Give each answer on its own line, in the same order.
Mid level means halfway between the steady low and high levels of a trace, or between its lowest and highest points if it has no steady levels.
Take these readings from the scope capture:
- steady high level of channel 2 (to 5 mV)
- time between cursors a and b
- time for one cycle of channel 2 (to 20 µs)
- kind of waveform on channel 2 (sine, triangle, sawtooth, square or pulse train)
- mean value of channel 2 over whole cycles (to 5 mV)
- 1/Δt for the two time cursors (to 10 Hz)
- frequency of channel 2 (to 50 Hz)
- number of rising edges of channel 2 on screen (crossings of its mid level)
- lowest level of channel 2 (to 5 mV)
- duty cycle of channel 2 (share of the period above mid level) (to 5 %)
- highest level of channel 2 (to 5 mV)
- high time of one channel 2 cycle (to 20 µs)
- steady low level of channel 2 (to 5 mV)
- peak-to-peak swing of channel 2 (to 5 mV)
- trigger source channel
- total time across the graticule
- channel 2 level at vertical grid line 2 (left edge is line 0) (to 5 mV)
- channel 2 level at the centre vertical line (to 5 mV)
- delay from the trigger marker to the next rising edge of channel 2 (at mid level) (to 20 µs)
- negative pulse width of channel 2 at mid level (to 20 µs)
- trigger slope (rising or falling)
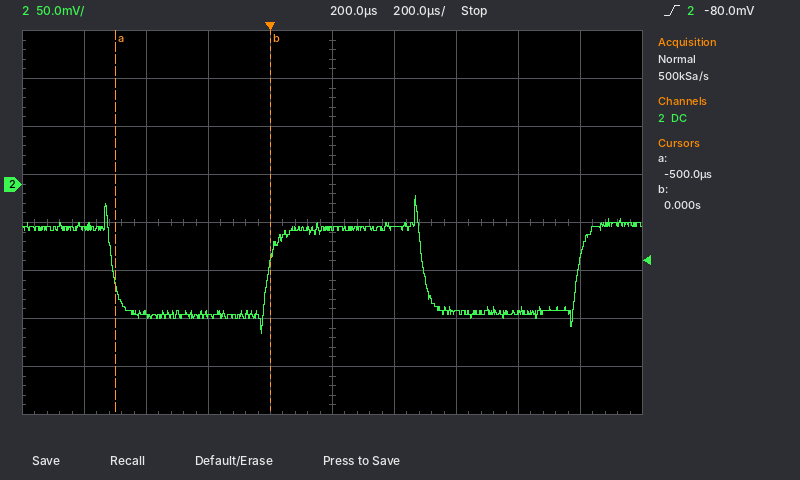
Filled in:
-45 mV
500 µs
1.00 ms
square
-90 mV
2.00 kHz
1.00 kHz
2
-155 mV
50 %
-10 mV
500 µs
-135 mV
145 mV
channel 2
2 ms
-135 mV
-45 mV
1.00 ms
500 µs
rising
